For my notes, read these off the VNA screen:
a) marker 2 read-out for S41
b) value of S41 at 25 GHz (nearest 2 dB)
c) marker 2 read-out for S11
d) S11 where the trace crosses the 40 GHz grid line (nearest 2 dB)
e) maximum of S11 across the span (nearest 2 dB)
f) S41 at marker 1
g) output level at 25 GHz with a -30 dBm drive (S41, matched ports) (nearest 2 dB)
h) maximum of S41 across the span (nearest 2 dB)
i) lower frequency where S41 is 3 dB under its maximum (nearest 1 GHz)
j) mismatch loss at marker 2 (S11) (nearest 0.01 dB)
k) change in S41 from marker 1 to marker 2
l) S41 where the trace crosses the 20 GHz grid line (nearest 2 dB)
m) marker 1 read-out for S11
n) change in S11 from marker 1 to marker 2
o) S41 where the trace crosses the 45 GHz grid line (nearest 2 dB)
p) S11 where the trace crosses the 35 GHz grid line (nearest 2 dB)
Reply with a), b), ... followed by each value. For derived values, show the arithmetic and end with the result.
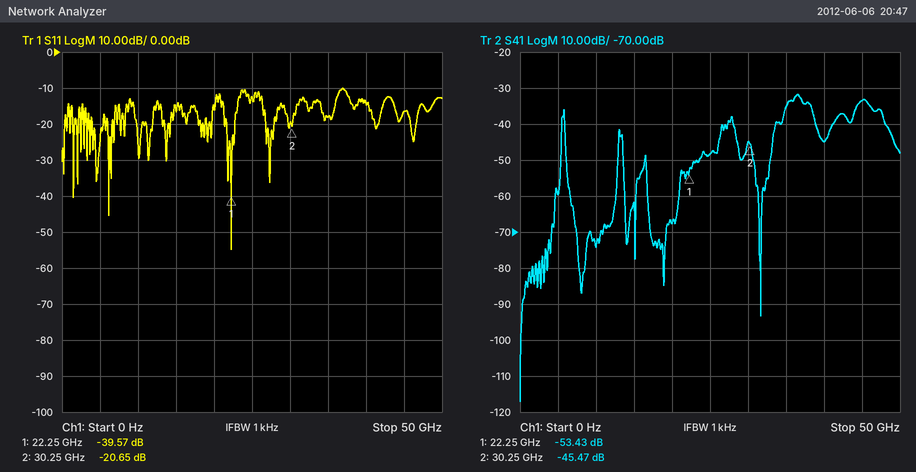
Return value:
a) -45.47 dB
b) -48 dB
c) -20.65 dB
d) -14 dB
e) -10 dB
f) -53.43 dB
g) -30 dBm + (-48 dB) = -78 dBm
h) -32 dB
i) 35 GHz
j) −10 log10(1 − 10^(-20.65/10)) ≈ 0.04 dB
k) -45.47 − (-53.43) = 7.96 dB
l) -68 dB
m) -39.57 dB
n) -20.65 − (-39.57) = 18.92 dB
o) -34 dB
p) -18 dB
